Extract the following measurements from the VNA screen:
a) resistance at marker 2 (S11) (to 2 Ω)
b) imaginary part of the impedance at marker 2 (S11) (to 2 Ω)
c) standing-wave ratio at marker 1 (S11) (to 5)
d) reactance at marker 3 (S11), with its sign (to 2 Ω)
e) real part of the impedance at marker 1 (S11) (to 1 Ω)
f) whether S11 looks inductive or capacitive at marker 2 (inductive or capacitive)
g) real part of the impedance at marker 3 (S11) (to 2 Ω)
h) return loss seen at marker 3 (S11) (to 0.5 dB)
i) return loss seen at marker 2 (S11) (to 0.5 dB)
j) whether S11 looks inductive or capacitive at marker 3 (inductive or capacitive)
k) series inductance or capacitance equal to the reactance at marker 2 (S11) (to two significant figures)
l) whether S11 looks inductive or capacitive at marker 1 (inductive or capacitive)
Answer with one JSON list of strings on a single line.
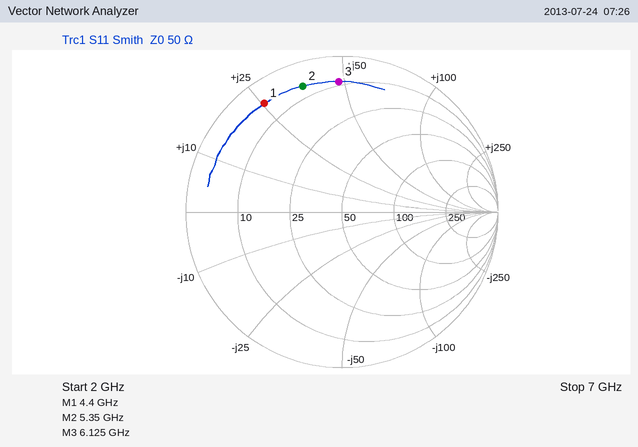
["6 Ω", "+36 Ω", "15", "+48 Ω", "5 Ω", "inductive", "8 Ω", "1.5 dB", "1.5 dB", "inductive", "1.1 nH", "inductive"]
